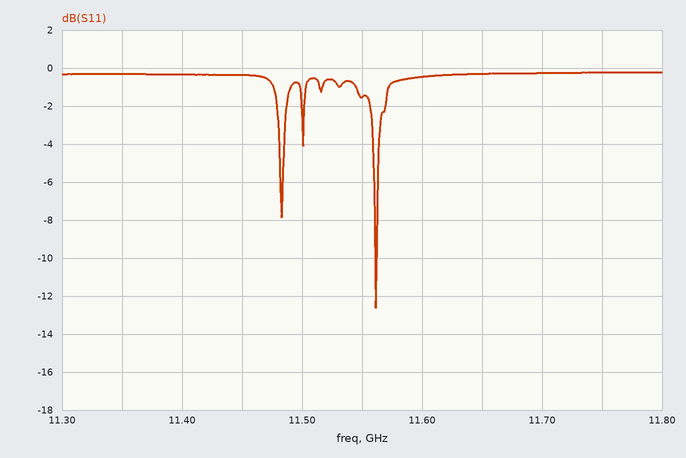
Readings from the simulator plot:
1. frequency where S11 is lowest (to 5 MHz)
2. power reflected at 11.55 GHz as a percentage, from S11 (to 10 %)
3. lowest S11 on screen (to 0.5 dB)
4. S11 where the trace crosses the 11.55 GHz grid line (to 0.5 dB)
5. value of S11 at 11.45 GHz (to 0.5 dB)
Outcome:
11.560 GHz
70 %
-12.5 dB
-1.5 dB
-0.5 dB
